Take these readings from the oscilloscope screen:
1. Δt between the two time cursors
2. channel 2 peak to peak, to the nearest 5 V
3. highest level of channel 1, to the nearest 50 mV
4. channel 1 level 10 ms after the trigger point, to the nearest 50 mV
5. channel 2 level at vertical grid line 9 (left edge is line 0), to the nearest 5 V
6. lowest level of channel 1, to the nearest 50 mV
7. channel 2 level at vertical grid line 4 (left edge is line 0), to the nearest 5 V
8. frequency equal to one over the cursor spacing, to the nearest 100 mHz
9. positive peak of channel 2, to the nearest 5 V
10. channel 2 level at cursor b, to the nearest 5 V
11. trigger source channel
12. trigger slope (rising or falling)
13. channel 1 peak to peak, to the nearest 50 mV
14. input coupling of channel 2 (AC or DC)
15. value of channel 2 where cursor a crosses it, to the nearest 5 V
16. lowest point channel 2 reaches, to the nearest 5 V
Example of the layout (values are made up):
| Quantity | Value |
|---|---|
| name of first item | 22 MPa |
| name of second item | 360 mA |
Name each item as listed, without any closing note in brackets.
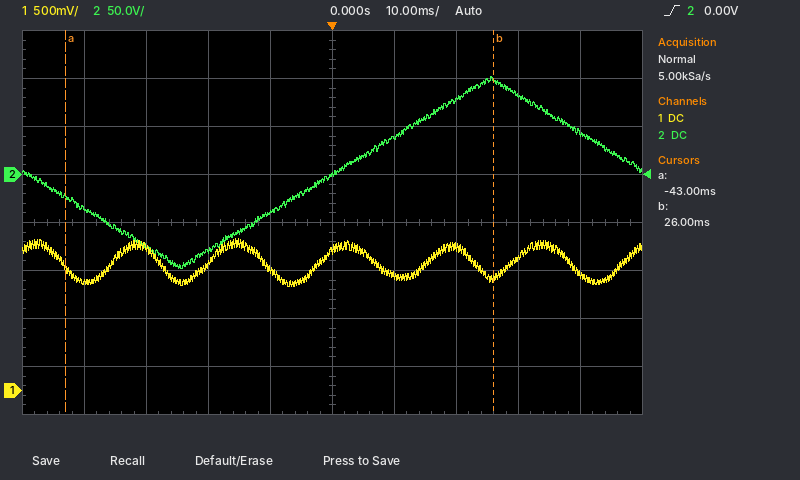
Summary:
| Quantity | Value |
|---|---|
| Δt between the two time cursors | 69 ms |
| channel 2 peak to peak, to the nearest 5 V | 200 V |
| highest level of channel 1, to the nearest 50 mV | 1.60 V |
| channel 1 level 10 ms after the trigger point, to the nearest 50 mV | 1.20 V |
| channel 2 level at vertical grid line 9 (left edge is line 0), to the nearest 5 V | 45 V |
| lowest level of channel 1, to the nearest 50 mV | 1.10 V |
| channel 2 level at vertical grid line 4 (left edge is line 0), to the nearest 5 V | -40 V |
| frequency equal to one over the cursor spacing, to the nearest 100 mHz | 14.5 Hz |
| positive peak of channel 2, to the nearest 5 V | 100 V |
| channel 2 level at cursor b, to the nearest 5 V | 100 V |
| trigger source channel | channel 2 |
| trigger slope | rising |
| channel 1 peak to peak, to the nearest 50 mV | 500 mV |
| input coupling of channel 2 | DC |
| value of channel 2 where cursor a crosses it, to the nearest 5 V | -25 V |
| lowest point channel 2 reaches, to the nearest 5 V | -100 V |
